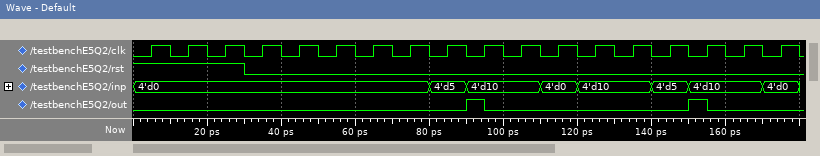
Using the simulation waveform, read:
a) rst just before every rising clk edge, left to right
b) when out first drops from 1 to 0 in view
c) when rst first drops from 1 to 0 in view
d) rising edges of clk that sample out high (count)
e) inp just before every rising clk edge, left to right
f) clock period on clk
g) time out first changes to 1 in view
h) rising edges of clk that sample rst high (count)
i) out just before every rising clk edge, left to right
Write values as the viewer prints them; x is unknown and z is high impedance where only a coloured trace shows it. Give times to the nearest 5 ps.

1 1 1 0 0 0 0 0 0 0 0 0 0 0 0 0 0 0
95 ps
30 ps
2
4'd0, 4'd0, 4'd0, 4'd0, 4'd0, 4'd0, 4'd0, 4'd0, 4'd5, 4'd10, 4'd10, 4'd0, 4'd10, 4'd10, 4'd5, 4'd10, 4'd10, 4'd0
10 ps
90 ps
3
0 0 0 0 0 0 0 0 0 1 0 0 0 0 0 1 0 0
